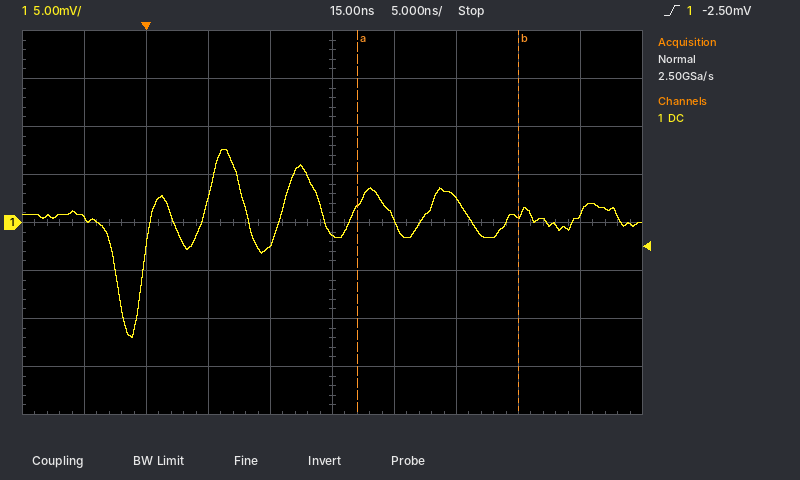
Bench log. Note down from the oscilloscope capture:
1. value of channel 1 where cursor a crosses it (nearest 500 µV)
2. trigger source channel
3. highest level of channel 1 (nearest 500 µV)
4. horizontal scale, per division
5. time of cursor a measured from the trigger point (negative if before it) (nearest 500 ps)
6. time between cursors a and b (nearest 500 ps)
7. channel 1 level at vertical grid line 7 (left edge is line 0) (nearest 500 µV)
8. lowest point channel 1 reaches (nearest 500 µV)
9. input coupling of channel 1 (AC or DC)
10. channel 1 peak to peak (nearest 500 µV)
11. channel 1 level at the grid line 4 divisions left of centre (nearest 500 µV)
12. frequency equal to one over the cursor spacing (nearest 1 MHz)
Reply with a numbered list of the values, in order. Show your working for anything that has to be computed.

1. 1.5 mV
2. channel 1
3. 7.5 mV
4. 5 ns
5. +17.0 ns
6. 13.0 ns
7. 2.5 mV
8. -12.0 mV
9. DC
10. 7.5 mV − (-12.0 mV) = 19.5 mV
11. 500 µV
12. 1 / 13.0 ns ≈ 77 MHz
